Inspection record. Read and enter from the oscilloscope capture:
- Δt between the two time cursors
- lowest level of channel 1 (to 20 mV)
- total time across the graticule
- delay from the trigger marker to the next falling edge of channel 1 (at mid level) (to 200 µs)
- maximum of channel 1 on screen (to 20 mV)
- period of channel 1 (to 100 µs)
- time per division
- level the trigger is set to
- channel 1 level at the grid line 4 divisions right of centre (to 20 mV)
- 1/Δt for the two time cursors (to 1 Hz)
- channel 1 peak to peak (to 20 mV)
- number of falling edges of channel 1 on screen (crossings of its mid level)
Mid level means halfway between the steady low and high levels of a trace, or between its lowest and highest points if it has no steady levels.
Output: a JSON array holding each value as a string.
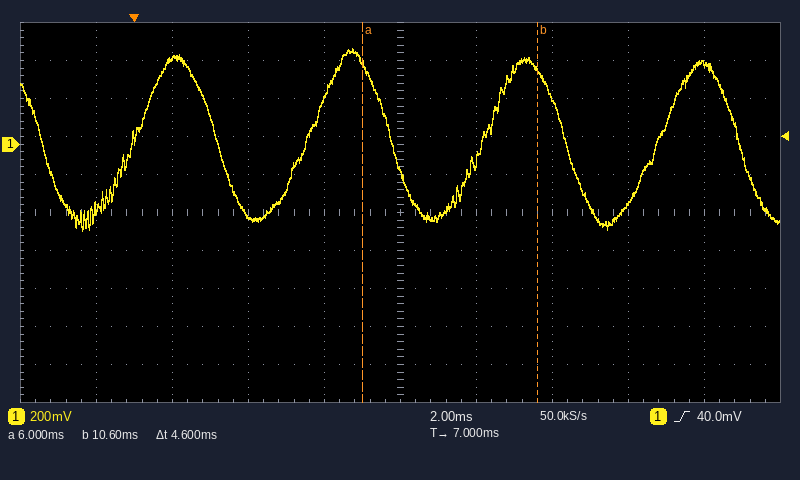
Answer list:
["4.6 ms", "-460 mV", "20 ms", "2.2 ms", "500 mV", "4.6 ms", "2 ms", "40.0 mV", "420 mV", "217 Hz", "960 mV", "5"]
